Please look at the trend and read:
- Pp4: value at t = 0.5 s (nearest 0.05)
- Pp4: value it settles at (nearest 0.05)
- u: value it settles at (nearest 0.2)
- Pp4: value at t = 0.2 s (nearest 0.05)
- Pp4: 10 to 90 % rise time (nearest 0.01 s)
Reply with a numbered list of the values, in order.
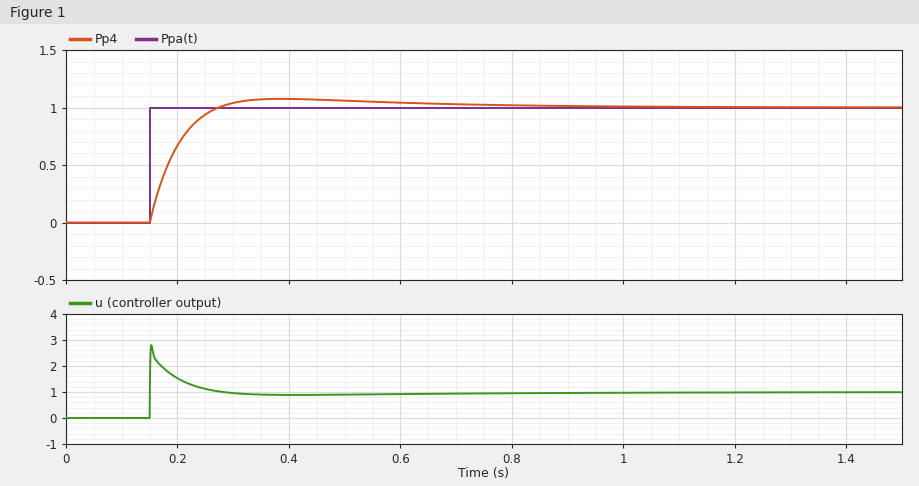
1. 1.05
2. 1.00
3. 1.0
4. 0.65
5. 0.08 s
